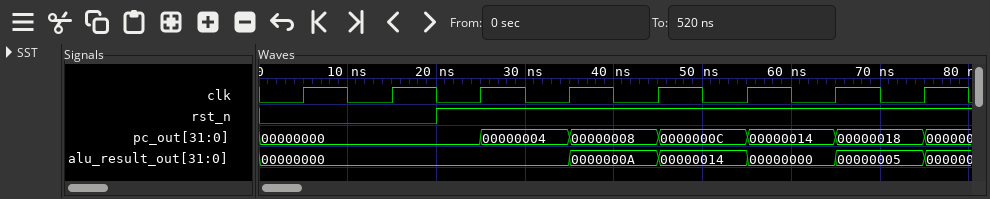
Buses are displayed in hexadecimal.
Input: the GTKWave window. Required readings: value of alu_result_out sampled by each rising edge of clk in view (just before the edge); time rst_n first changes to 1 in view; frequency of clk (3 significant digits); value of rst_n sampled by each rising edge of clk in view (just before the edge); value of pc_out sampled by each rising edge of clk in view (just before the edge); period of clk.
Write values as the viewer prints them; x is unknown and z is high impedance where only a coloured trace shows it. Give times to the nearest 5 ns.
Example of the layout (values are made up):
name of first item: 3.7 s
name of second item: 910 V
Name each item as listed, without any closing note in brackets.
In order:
value of alu_result_out sampled by each rising edge of clk in view: 00000000, 00000000, 00000000, 00000000, 0000000A, 00000014, 00000000, 00000005
time rst_n first changes to 1 in view: 20 ns
frequency of clk: 100 MHz
value of rst_n sampled by each rising edge of clk in view: 0 0 1 1 1 1 1 1
value of pc_out sampled by each rising edge of clk in view: 00000000, 00000000, 00000000, 00000004, 00000008, 0000000C, 00000014, 00000018
period of clk: 10 ns
